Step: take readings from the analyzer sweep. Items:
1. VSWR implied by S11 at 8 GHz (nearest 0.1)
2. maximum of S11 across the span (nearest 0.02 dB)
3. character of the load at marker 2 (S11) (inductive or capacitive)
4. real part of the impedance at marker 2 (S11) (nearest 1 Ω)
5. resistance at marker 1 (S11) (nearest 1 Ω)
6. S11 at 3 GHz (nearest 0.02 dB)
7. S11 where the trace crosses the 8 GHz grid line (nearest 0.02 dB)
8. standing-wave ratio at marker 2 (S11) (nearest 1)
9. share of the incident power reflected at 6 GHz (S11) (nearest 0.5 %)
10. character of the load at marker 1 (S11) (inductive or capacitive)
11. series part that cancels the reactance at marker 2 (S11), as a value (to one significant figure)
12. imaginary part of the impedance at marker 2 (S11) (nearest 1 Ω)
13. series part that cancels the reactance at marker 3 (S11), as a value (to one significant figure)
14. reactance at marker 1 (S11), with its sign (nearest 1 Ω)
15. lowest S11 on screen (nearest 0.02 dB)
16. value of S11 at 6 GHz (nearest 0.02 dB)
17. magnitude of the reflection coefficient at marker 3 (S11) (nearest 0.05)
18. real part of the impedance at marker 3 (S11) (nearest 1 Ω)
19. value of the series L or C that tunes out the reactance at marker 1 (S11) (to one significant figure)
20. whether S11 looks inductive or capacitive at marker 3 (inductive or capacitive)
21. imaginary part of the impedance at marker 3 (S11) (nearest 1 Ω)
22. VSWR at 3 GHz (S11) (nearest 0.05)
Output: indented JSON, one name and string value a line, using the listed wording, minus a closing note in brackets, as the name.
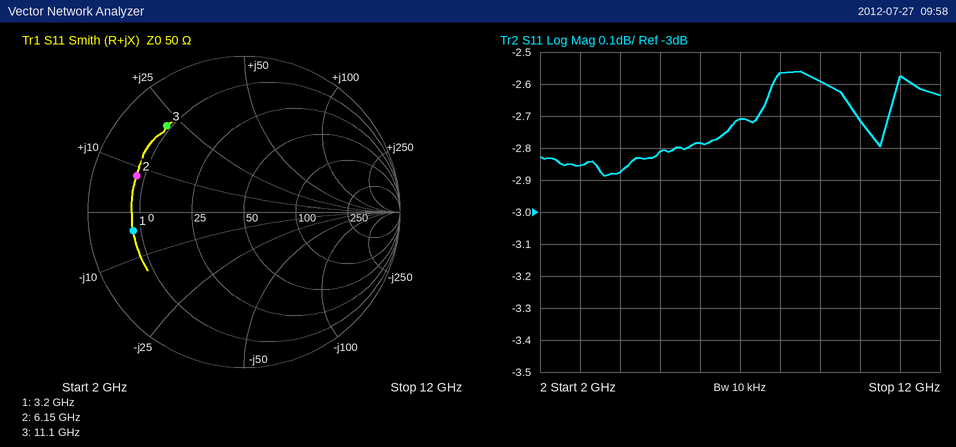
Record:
{
  "VSWR implied by S11 at 8 GHz": "6.8",
  "maximum of S11 across the span": "-2.56 dB",
  "character of the load at marker 2 (S11)": "inductive",
  "real part of the impedance at marker 2 (S11)": "8 Ω",
  "resistance at marker 1 (S11)": "8 Ω",
  "S11 at 3 GHz": "-2.86 dB",
  "S11 where the trace crosses the 8 GHz grid line": "-2.56 dB",
  "standing-wave ratio at marker 2 (S11)": "6",
  "share of the incident power reflected at 6 GHz (S11)": "52.5 %",
  "character of the load at marker 1 (S11)": "capacitive",
  "series part that cancels the reactance at marker 2 (S11), as a value": "3 pF",
  "imaginary part of the impedance at marker 2 (S11)": "+8 Ω",
  "series part that cancels the reactance at marker 3 (S11), as a value": "700 fF",
  "reactance at marker 1 (S11), with its sign": "-4 Ω",
  "lowest S11 on screen": "-2.88 dB",
  "value of S11 at 6 GHz": "-2.78 dB",
  "magnitude of the reflection coefficient at marker 3 (S11)": "0.75",
  "real part of the impedance at marker 3 (S11)": "9 Ω",
  "value of the series L or C that tunes out the reactance at marker 1 (S11)": "200 pH",
  "whether S11 looks inductive or capacitive at marker 3": "inductive",
  "imaginary part of the impedance at marker 3 (S11)": "+22 Ω",
  "VSWR at 3 GHz (S11)": "6.15"
}
